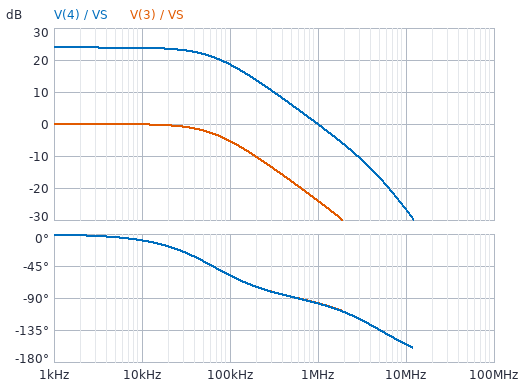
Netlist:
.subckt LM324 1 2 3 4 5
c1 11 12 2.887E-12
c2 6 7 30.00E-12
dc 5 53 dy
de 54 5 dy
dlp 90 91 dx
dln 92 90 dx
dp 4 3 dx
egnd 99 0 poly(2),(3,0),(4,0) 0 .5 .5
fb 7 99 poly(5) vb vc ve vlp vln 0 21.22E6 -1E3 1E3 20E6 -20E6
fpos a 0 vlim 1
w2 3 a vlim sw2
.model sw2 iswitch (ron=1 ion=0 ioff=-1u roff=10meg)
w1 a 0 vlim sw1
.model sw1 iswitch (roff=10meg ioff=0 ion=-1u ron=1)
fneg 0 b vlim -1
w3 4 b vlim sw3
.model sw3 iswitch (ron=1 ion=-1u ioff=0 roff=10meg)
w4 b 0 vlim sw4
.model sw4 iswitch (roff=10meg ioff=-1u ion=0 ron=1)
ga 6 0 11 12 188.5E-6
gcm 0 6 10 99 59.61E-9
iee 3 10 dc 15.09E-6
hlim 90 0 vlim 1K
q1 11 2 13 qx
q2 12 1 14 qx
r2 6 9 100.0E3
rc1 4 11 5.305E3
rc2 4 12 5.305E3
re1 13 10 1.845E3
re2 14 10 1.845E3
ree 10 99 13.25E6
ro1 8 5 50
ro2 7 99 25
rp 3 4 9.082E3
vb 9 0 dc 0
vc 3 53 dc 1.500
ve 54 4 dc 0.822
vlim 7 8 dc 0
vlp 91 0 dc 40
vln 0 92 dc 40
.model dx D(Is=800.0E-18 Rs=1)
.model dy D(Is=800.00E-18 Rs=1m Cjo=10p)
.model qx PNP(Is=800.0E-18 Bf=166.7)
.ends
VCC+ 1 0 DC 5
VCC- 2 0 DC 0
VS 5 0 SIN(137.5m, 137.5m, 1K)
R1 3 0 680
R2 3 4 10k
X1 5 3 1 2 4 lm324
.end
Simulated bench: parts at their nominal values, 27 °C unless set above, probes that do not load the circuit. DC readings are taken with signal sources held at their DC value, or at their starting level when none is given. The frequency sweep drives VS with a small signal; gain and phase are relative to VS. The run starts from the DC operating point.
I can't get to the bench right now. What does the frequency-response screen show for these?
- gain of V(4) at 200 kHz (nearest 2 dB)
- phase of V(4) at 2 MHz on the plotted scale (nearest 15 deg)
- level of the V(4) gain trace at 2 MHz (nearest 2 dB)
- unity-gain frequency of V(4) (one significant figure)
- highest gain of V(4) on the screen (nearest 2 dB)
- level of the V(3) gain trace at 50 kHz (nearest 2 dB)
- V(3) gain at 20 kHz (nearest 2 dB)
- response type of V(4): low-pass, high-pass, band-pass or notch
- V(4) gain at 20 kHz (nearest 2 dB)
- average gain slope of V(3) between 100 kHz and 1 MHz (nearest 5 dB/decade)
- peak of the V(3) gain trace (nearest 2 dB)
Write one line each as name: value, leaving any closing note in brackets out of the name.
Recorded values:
gain of V(4) at 200 kHz: 14 dB
phase of V(4) at 2 MHz on the plotted scale: -105 deg
level of the V(4) gain trace at 2 MHz: -6 dB
unity-gain frequency of V(4): 1 MHz
highest gain of V(4) on the screen: 24 dB
level of the V(3) gain trace at 50 kHz: -2 dB
V(3) gain at 20 kHz: 0 dB
response type of V(4): low-pass, high-pass, band-pass or notch: low-pass
V(4) gain at 20 kHz: 24 dB
average gain slope of V(3) between 100 kHz and 1 MHz: -20 dB/decade
peak of the V(3) gain trace: 0 dB
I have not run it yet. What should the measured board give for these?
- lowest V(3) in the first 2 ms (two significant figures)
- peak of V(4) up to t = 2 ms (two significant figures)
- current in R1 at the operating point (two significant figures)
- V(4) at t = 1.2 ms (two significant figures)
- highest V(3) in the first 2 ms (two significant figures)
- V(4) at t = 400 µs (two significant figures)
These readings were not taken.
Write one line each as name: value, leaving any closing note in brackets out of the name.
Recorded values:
lowest V(3) in the first 2 ms: 3.1 mV
peak of V(4) up to t = 2 ms: 4.3 V
current in R1 at the operating point: 200 µA
V(4) at t = 1.2 ms: 4.2 V
highest V(3) in the first 2 ms: 270 mV
V(4) at t = 400 µs: 3.5 V
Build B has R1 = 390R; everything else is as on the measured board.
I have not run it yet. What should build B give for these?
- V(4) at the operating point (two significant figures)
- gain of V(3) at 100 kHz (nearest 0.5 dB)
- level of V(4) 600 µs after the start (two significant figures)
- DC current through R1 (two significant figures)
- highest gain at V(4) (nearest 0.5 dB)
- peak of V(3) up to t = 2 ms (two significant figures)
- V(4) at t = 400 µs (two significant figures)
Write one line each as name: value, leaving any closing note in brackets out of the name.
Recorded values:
V(4) at the operating point: 3.7 V
gain of V(3) at 100 kHz: -9.0 dB
level of V(4) 600 µs after the start: 1.6 V
DC current through R1: 350 µA
highest gain at V(4): 28.5 dB
peak of V(3) up to t = 2 ms: 160 mV
V(4) at t = 400 µs: 4.3 V
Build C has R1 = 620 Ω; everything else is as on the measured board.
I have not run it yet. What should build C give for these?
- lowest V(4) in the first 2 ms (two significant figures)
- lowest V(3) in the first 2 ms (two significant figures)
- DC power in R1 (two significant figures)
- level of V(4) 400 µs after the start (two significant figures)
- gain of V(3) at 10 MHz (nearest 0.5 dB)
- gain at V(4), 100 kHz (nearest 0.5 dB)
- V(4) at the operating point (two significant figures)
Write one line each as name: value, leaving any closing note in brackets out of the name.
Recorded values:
lowest V(4) in the first 2 ms: 51 mV
lowest V(3) in the first 2 ms: 3.0 mV
DC power in R1: 31 µW
level of V(4) 400 µs after the start: 3.8 V
gain of V(3) at 10 MHz: -52.5 dB
gain at V(4), 100 kHz: 19.0 dB
V(4) at the operating point: 2.4 V
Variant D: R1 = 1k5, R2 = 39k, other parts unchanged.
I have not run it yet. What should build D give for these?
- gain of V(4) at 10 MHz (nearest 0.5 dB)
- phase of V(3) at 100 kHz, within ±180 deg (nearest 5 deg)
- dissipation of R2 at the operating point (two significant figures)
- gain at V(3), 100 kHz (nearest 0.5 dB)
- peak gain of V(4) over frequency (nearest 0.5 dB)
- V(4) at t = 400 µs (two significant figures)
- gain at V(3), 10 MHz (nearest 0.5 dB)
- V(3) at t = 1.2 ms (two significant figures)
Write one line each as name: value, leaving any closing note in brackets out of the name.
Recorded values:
gain of V(4) at 10 MHz: -26.5 dB
phase of V(3) at 100 kHz, within ±180 deg: -70 deg
dissipation of R2 at the operating point: 330 µW
gain at V(3), 100 kHz: -9.0 dB
peak gain of V(4) over frequency: 28.5 dB
V(4) at t = 400 µs: 4.3 V
gain at V(3), 10 MHz: -60.0 dB
V(3) at t = 1.2 ms: 160 mV
